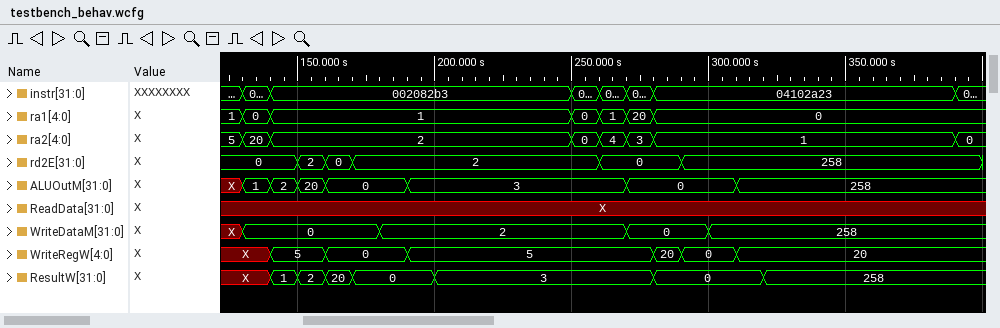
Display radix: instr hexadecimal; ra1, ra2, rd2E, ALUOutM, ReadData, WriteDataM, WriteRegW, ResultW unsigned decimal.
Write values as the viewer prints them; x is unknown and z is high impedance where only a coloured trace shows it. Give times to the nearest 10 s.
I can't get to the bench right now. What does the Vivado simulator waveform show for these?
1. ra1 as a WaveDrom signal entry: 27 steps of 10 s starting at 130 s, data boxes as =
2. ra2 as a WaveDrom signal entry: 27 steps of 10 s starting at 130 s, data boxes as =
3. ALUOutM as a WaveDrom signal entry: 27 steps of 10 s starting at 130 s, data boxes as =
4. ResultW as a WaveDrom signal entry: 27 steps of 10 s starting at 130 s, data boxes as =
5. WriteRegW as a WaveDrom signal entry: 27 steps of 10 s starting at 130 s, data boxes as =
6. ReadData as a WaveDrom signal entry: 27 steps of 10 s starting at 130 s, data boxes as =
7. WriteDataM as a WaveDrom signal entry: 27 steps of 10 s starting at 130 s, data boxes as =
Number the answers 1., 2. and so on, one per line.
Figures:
1. {name: 'ra1', wave: '==..........====...........', data: '0 1 0 1 20 0'}
2. {name: 'ra2', wave: '==..........====..........=', data: '20 2 0 4 3 1 0'}
3. {name: 'ALUOutM', wave: '====..=.......=...=........', data: '1 2 20 0 3 0 258'}
4. {name: 'ResultW', wave: 'x====..=.......=...=.......', data: '1 2 20 0 3 0 258'}
5. {name: 'WriteRegW', wave: 'x=.=..=........==.=........', data: '5 0 5 20 0 20'}
6. {name: 'ReadData', wave: 'x..........................'}
7. {name: 'WriteDataM', wave: '=....=........=..=.........', data: '0 2 0 258'}
